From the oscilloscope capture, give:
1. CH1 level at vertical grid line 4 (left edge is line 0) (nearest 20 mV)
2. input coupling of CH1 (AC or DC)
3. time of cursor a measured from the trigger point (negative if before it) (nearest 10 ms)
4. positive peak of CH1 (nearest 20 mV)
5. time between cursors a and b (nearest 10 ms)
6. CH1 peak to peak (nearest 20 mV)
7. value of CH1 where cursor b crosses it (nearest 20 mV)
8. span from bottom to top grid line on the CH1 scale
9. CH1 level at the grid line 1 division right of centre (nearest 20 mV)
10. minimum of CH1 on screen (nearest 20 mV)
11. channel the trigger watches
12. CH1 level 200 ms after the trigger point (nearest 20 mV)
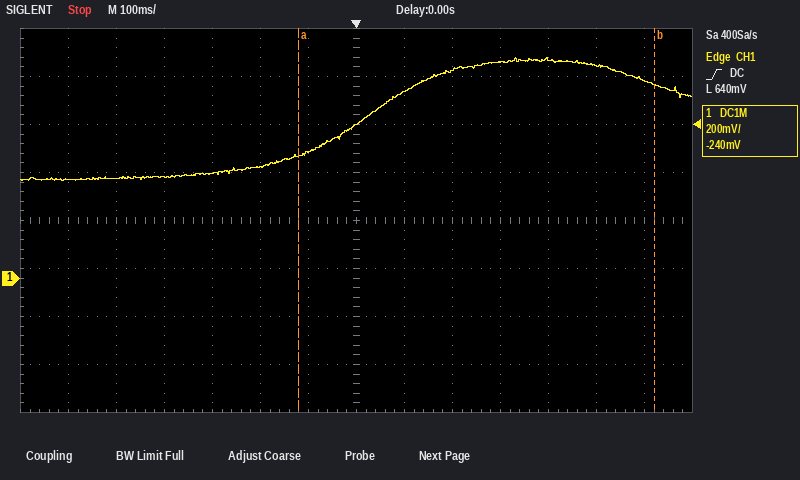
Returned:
440 mV
DC
-120 ms
920 mV
740 ms
520 mV
800 mV
1.6 V
780 mV
400 mV
CH1
860 mV
